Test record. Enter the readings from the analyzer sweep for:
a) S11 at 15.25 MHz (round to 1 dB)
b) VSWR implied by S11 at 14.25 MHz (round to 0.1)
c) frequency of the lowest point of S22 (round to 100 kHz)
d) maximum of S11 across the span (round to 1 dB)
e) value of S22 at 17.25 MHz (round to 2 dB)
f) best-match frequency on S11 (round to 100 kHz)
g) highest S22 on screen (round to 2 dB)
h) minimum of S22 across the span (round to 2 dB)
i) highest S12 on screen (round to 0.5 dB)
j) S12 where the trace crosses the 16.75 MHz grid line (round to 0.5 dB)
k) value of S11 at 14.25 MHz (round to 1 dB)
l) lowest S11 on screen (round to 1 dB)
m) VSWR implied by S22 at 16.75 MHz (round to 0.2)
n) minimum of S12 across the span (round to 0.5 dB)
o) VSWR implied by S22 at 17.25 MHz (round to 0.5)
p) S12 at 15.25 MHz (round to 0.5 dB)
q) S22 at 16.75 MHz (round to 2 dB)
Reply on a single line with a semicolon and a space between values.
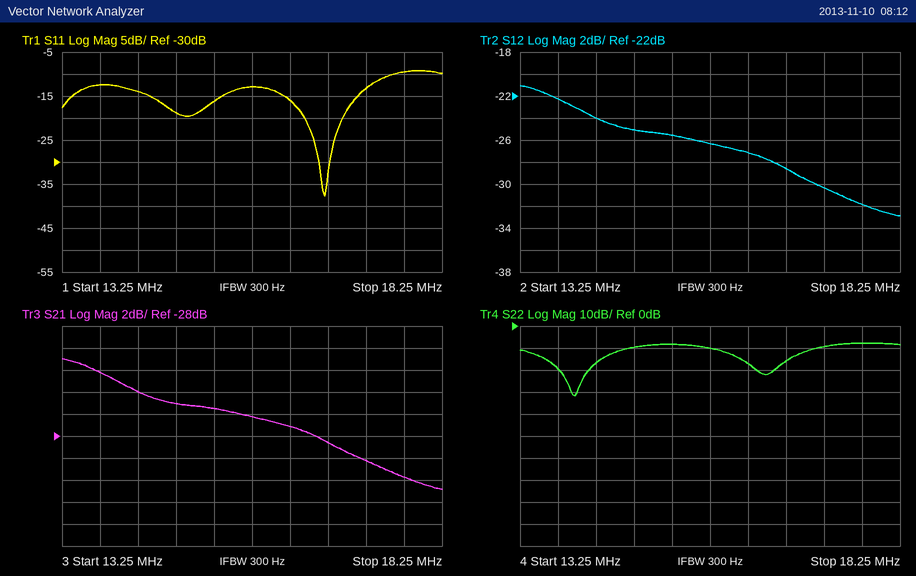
-16 dB; 1.5; 14.0 MHz; -9 dB; -10 dB; 16.7 MHz; -8 dB; -32 dB; -21.0 dB; -28.5 dB; -14 dB; -38 dB; 1.4; -33.0 dB; 2.0; -25.5 dB; -16 dB
